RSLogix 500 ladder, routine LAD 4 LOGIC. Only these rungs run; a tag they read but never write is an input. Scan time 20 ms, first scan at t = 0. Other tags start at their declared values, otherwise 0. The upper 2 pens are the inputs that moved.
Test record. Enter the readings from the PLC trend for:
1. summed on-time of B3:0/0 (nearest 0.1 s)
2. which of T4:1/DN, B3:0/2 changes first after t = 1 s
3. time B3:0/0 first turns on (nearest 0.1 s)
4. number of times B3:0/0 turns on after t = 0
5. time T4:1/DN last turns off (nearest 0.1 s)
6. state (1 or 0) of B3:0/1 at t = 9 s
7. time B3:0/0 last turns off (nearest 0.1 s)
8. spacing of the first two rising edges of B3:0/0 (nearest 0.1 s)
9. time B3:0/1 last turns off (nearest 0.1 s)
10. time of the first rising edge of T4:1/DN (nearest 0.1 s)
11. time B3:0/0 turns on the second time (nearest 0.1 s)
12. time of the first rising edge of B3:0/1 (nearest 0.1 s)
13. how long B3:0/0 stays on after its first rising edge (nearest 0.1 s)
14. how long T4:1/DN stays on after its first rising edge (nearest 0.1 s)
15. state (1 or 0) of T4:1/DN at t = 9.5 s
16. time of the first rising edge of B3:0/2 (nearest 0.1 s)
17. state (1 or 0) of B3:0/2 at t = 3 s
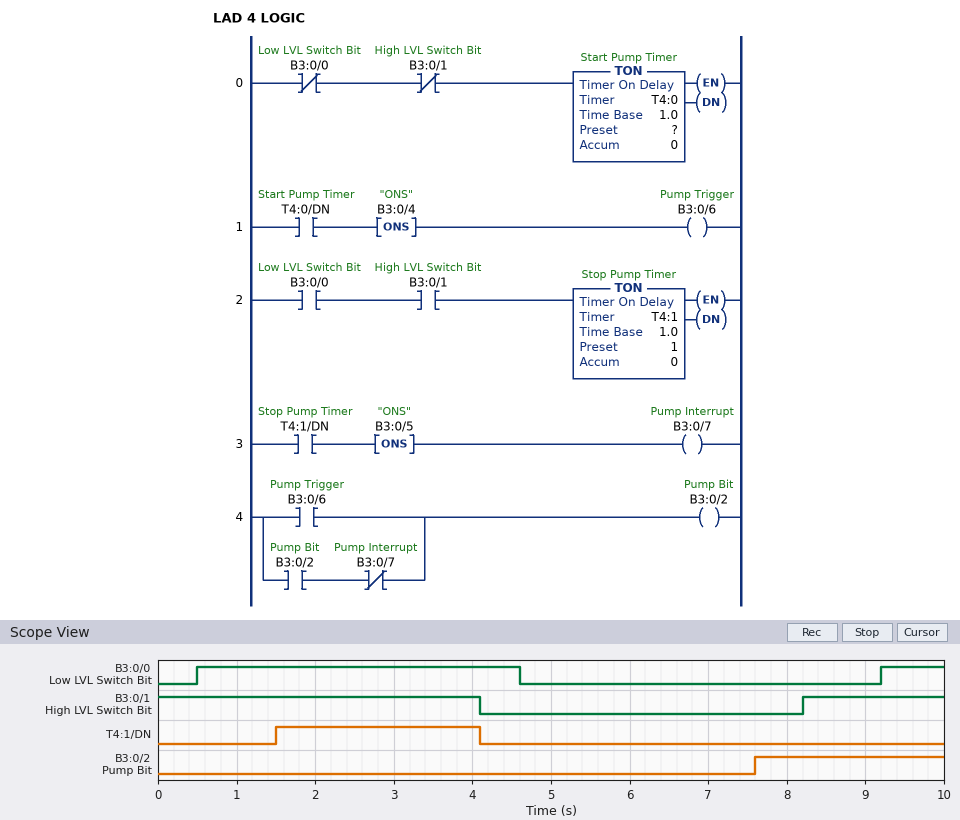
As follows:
4.9 s
T4:1/DN
0.5 s
2
4.1 s
1
4.6 s
8.7 s
4.1 s
1.5 s
9.2 s
8.2 s
4.1 s
2.6 s
0
7.6 s
0
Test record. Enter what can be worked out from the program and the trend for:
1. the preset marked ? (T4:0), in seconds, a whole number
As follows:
3 s
